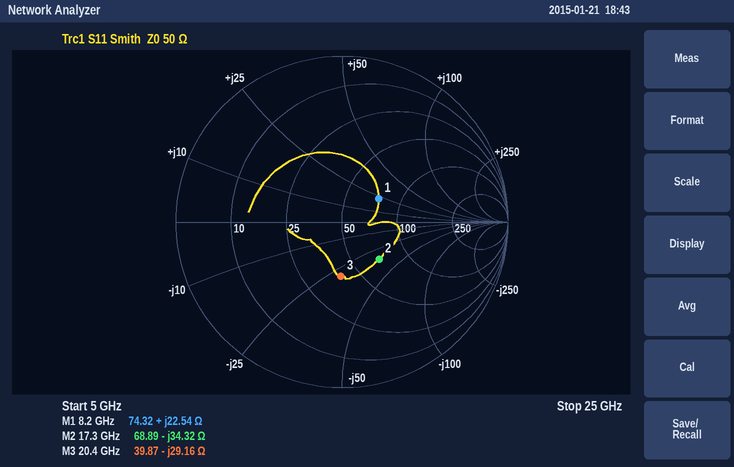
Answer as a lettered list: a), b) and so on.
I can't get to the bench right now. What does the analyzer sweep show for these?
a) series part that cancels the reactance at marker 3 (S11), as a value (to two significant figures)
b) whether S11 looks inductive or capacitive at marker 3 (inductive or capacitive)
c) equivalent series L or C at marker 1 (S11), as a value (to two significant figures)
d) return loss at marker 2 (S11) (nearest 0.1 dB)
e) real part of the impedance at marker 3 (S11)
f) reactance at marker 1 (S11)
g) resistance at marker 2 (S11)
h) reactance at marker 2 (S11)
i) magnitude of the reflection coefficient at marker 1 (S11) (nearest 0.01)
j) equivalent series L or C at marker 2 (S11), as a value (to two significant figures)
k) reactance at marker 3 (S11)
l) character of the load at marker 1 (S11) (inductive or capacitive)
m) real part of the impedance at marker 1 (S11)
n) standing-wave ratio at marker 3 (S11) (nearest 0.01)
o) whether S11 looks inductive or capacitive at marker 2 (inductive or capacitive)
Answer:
a) 230 pH
b) capacitive
c) 440 pH
d) 10.0 dB
e) 39.87 Ω
f) +22.54 Ω
g) 68.89 Ω
h) -34.32 Ω
i) 0.26
j) 270 fF
k) -29.16 Ω
l) inductive
m) 74.32 Ω
n) 1.97
o) capacitive
